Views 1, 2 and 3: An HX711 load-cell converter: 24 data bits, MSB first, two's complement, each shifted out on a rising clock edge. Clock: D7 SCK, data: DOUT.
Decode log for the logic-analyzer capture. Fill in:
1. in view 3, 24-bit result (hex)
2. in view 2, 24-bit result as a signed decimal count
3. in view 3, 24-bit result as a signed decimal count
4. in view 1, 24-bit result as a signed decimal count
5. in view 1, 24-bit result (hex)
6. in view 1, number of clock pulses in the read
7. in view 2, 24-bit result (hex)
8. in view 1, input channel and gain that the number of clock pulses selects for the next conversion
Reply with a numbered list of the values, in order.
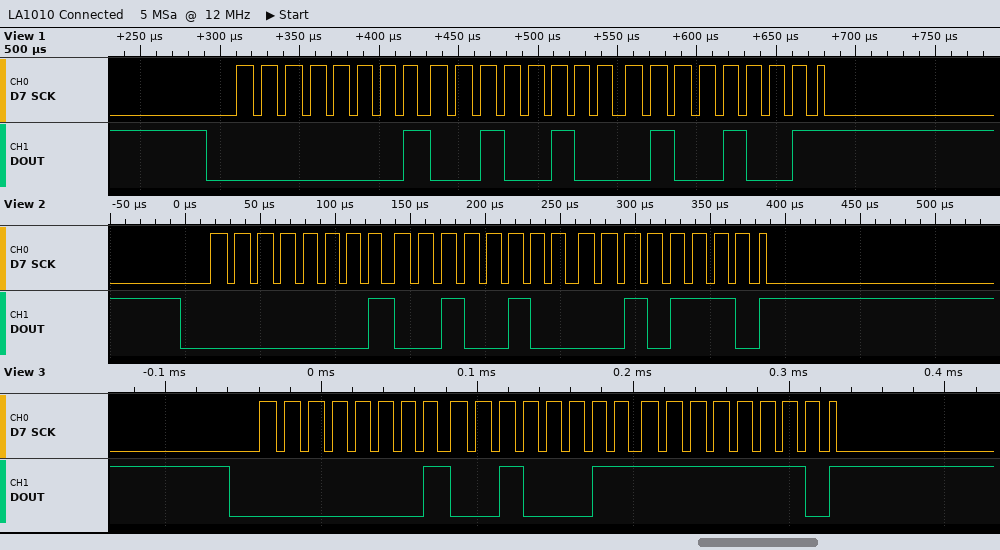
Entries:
1. 0x0123FE
2. 74798
3. 74750
4. 74825
5. 0x012449
6. 25
7. 0x01242E
8. channel A, gain 128
